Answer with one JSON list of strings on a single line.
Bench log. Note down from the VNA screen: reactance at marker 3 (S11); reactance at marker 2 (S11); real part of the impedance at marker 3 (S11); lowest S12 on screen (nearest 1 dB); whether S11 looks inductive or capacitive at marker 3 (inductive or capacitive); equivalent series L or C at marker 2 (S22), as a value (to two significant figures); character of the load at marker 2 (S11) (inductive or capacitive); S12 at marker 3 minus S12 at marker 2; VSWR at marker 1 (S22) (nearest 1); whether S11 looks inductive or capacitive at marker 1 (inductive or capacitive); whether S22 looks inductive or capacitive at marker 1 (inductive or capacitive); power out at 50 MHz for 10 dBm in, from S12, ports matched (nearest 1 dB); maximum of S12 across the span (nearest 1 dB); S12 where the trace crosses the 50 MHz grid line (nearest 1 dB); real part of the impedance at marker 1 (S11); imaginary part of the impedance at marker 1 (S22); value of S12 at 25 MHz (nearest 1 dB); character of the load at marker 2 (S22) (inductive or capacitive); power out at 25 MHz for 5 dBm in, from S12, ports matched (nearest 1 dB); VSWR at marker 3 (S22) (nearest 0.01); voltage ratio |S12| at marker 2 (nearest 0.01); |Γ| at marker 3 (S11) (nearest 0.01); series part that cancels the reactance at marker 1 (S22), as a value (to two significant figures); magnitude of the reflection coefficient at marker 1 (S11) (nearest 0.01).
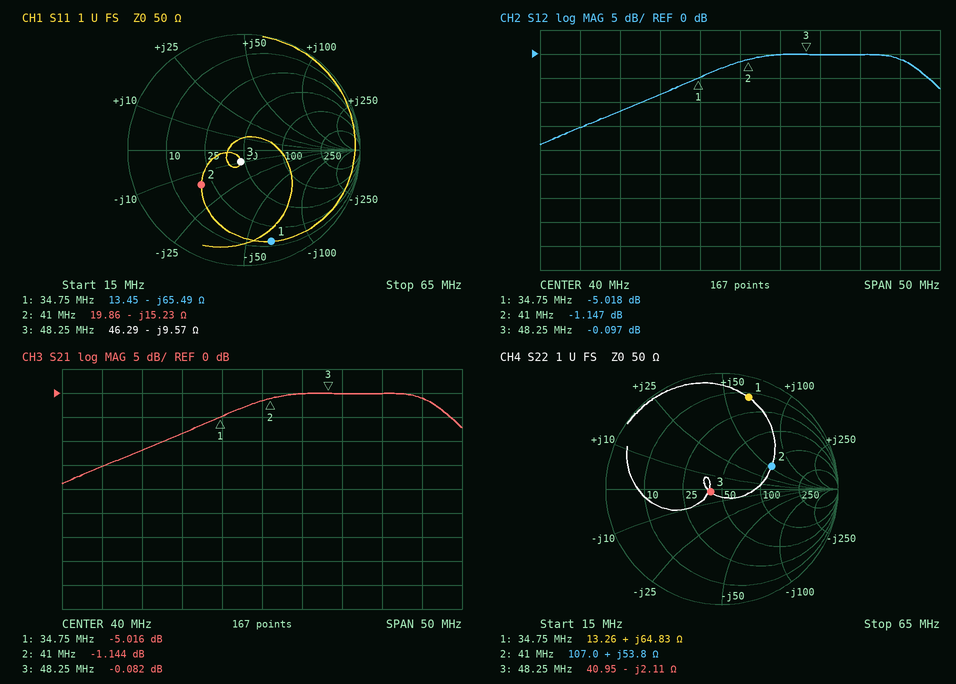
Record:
["-9.57 Ω", "-15.23 Ω", "46.29 Ω", "-19 dB", "capacitive", "210 nH", "capacitive", "1.050 dB", "10", "capacitive", "inductive", "10 dBm", "0 dB", "0 dB", "13.45 Ω", "+64.83 Ω", "-12 dB", "inductive", "-7 dBm", "1.23", "0.88", "0.11", "71 pF", "0.82"]
